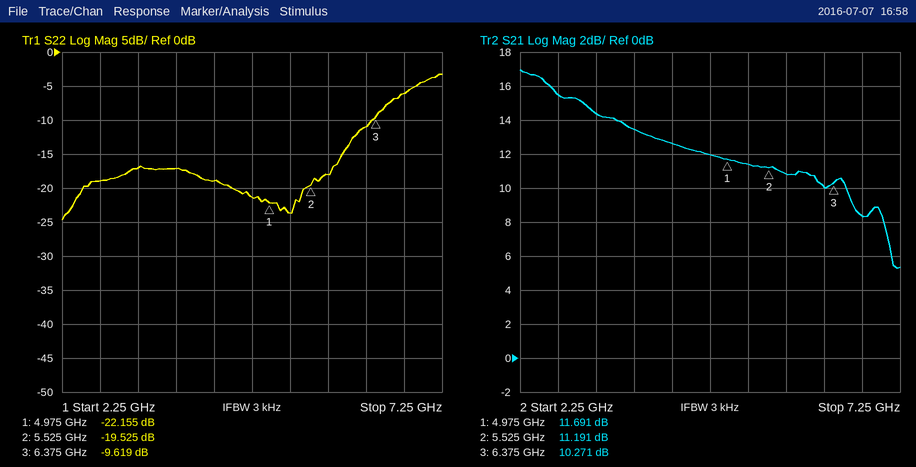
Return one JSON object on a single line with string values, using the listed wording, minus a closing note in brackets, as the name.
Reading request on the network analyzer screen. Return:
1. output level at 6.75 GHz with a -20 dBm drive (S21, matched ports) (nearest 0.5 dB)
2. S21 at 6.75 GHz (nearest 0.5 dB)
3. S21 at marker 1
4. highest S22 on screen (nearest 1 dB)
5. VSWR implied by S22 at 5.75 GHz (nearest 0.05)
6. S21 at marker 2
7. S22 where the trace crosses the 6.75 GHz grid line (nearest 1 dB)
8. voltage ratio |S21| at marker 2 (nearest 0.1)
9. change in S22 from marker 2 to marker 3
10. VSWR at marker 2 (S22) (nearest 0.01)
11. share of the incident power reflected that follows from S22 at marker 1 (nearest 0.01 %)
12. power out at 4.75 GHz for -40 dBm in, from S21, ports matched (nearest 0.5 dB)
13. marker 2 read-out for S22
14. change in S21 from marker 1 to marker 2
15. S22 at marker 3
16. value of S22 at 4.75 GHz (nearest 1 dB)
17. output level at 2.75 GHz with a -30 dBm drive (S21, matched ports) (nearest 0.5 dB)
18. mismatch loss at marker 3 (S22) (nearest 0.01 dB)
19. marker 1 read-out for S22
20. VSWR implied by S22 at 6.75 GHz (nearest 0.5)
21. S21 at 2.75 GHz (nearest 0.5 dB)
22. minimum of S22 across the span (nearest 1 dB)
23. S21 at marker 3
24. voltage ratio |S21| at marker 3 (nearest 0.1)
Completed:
{"output level at 6.75 GHz with a -20 dBm drive (S21, matched ports)": "-11.5 dBm", "S21 at 6.75 GHz": "8.5 dB", "S21 at marker 1": "11.691 dB", "highest S22 on screen": "-3 dB", "VSWR implied by S22 at 5.75 GHz": "1.30", "S21 at marker 2": "11.191 dB", "S22 where the trace crosses the 6.75 GHz grid line": "-6 dB", "voltage ratio |S21| at marker 2": "3.6", "change in S22 from marker 2 to marker 3": "9.906 dB", "VSWR at marker 2 (S22)": "1.24", "share of the incident power reflected that follows from S22 at marker 1": "0.61 %", "power out at 4.75 GHz for -40 dBm in, from S21, ports matched": "-28.0 dBm", "marker 2 read-out for S22": "-19.525 dB", "change in S21 from marker 1 to marker 2": "-0.500 dB", "S22 at marker 3": "-9.619 dB", "value of S22 at 4.75 GHz": "-21 dB", "output level at 2.75 GHz with a -30 dBm drive (S21, matched ports)": "-14.5 dBm", "mismatch loss at marker 3 (S22)": "0.50 dB", "marker 1 read-out for S22": "-22.155 dB", "VSWR implied by S22 at 6.75 GHz": "3.0", "S21 at 2.75 GHz": "15.5 dB", "minimum of S22 across the span": "-25 dB", "S21 at marker 3": "10.271 dB", "voltage ratio |S21| at marker 3": "3.3"}
